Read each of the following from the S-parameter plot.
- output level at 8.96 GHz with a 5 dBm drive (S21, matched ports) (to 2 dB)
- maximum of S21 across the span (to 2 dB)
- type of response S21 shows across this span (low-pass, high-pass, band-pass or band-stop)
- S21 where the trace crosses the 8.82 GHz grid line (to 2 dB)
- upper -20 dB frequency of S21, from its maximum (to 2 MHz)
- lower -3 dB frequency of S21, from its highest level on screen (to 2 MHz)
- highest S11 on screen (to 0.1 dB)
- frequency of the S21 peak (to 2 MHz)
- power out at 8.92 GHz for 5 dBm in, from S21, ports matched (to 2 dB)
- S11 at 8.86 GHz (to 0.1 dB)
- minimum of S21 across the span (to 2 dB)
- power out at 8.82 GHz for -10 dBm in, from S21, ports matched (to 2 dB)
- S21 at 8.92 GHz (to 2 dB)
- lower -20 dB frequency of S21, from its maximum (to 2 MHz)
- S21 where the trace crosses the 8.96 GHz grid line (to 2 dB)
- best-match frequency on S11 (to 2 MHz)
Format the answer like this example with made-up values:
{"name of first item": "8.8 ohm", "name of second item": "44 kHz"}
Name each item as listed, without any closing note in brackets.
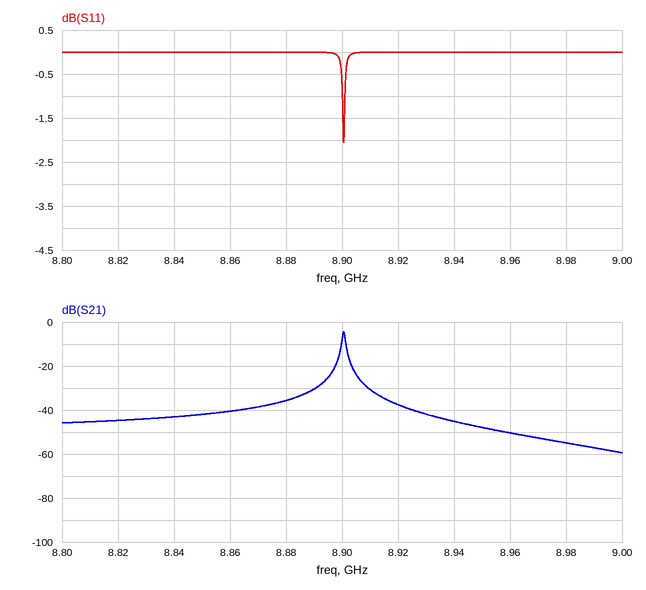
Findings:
{"output level at 8.96 GHz with a 5 dBm drive (S21, matched ports)": "-46 dBm", "maximum of S21 across the span": "-4 dB", "type of response S21 shows across this span": "band-pass", "S21 where the trace crosses the 8.82 GHz grid line": "-44 dB", "upper -20 dB frequency of S21, from its maximum": "8.906 GHz", "lower -3 dB frequency of S21, from its highest level on screen": "8.900 GHz", "highest S11 on screen": "0.0 dB", "frequency of the S21 peak": "8.900 GHz", "power out at 8.92 GHz for 5 dBm in, from S21, ports matched": "-32 dBm", "S11 at 8.86 GHz": "0.0 dB", "minimum of S21 across the span": "-60 dB", "power out at 8.82 GHz for -10 dBm in, from S21, ports matched": "-54 dBm", "S21 at 8.92 GHz": "-38 dB", "lower -20 dB frequency of S21, from its maximum": "8.896 GHz", "S21 where the trace crosses the 8.96 GHz grid line": "-50 dB", "best-match frequency on S11": "8.900 GHz"}
